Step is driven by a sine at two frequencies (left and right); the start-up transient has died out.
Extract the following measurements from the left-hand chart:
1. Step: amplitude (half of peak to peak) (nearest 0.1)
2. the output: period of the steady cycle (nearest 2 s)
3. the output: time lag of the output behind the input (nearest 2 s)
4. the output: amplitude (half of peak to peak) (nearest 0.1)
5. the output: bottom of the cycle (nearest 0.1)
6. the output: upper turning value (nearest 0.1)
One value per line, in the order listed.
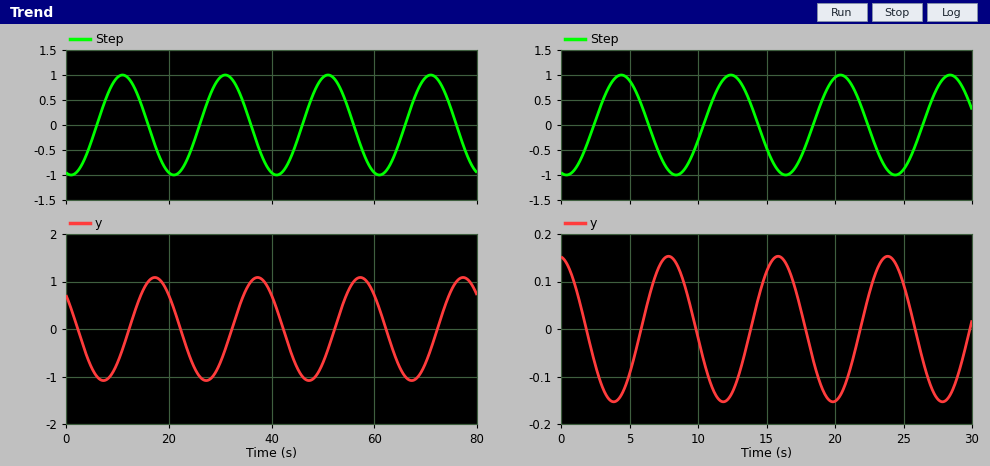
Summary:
1.0
20 s
6 s
1.1
-1.1
1.1
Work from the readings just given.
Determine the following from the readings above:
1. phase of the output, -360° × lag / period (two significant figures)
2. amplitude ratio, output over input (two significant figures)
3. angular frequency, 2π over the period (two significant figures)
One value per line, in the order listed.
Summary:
-110°
1.1
0.31 rad/s
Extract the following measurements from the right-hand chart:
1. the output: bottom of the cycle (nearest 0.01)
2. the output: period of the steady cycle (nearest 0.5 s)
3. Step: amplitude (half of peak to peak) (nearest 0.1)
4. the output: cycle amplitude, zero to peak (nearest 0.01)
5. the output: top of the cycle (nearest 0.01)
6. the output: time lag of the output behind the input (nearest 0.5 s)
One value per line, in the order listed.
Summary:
-0.15
8.0 s
1.0
0.15
0.15
3.5 s
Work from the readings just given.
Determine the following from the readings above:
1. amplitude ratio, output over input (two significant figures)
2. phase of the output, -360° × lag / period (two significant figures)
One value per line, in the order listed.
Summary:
0.15
-160°
